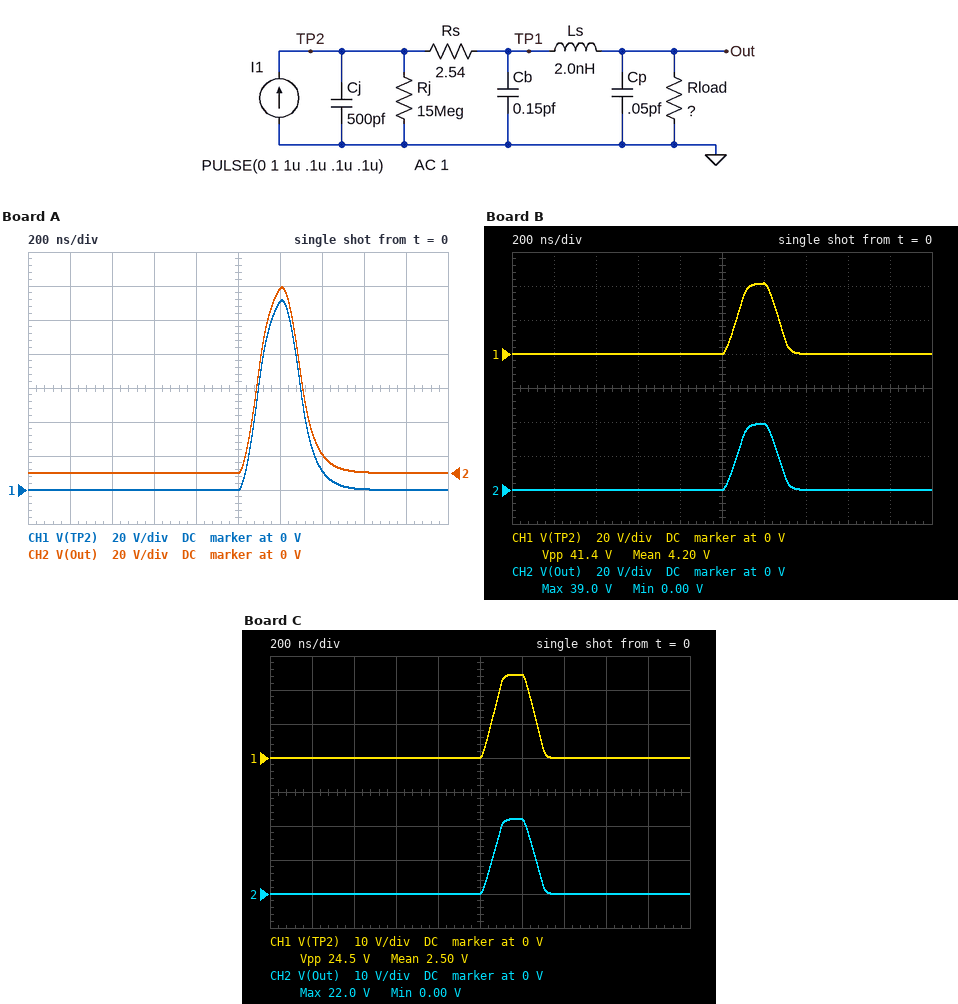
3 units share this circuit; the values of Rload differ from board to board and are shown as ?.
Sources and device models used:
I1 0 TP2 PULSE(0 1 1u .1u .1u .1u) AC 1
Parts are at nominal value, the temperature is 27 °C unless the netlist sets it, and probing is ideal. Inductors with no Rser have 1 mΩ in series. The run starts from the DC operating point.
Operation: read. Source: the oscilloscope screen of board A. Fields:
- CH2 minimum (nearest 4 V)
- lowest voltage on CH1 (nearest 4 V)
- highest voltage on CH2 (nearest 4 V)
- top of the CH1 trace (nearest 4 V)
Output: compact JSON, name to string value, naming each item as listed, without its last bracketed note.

{"CH2 minimum": "0 V", "lowest voltage on CH1": "0 V", "highest voltage on CH2": "108 V", "top of the CH1 trace": "112 V"}
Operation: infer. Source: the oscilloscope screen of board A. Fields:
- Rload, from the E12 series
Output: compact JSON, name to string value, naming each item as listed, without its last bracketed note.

{"Rload, from the E12 series": "120 Ω"}
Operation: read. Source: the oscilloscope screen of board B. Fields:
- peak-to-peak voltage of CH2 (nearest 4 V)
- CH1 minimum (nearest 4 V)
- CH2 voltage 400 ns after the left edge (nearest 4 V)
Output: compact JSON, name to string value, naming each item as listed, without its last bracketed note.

{"peak-to-peak voltage of CH2": "40 V", "CH1 minimum": "0 V", "CH2 voltage 400 ns after the left edge": "0 V"}
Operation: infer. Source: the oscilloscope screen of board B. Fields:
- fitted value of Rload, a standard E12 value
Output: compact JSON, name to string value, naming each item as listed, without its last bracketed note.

{"fitted value of Rload, a standard E12 value": "39 Ω"}
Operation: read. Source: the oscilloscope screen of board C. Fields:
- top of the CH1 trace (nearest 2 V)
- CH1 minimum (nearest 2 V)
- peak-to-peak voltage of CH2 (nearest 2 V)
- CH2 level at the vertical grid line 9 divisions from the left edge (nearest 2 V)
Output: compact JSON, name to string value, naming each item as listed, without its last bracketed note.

{"top of the CH1 trace": "24 V", "CH1 minimum": "0 V", "peak-to-peak voltage of CH2": "22 V", "CH2 level at the vertical grid line 9 divisions from the left edge": "0 V"}
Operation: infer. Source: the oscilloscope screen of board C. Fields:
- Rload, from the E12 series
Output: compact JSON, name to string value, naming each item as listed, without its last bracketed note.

{"Rload, from the E12 series": "22 Ω"}
